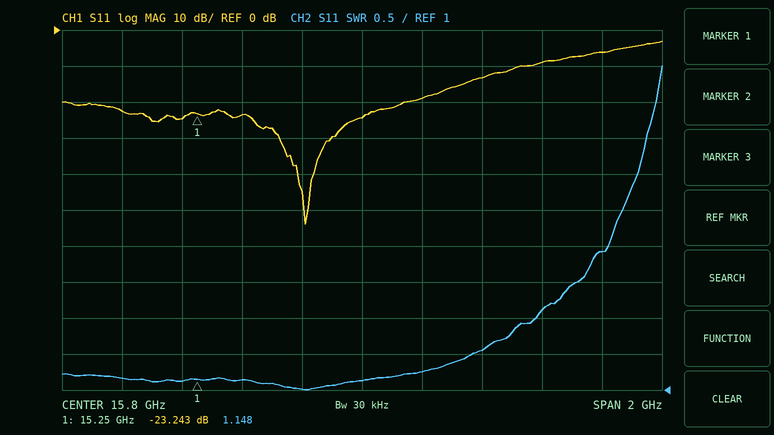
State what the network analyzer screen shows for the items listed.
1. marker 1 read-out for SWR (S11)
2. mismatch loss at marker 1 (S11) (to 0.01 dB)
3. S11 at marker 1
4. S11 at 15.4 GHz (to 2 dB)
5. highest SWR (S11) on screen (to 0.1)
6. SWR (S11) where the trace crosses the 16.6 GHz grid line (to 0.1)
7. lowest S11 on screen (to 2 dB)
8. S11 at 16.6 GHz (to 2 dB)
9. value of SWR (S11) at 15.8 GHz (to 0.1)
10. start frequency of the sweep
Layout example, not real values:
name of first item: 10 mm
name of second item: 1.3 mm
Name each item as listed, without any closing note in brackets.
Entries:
marker 1 read-out for SWR: 1.148
mismatch loss at marker 1 (S11): 0.02 dB
S11 at marker 1: -23.243 dB
S11 at 15.4 GHz: -24 dB
highest SWR (S11) on screen: 5.5
SWR (S11) where the trace crosses the 16.6 GHz grid line: 2.9
lowest S11 on screen: -54 dB
S11 at 16.6 GHz: -6 dB
value of SWR (S11) at 15.8 GHz: 1.1
start frequency of the sweep: 14.8 GHz
